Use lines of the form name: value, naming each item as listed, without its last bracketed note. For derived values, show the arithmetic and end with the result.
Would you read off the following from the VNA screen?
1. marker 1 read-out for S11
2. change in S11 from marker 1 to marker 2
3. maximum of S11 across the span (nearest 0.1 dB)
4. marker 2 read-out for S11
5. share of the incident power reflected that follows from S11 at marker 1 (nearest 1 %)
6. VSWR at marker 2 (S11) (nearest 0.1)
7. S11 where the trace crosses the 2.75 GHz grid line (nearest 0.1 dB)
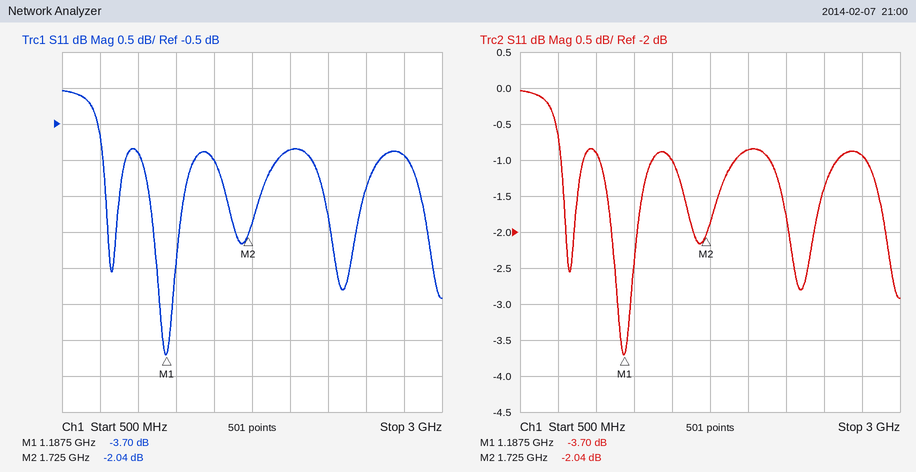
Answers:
marker 1 read-out for S11: -3.70 dB
change in S11 from marker 1 to marker 2: -2.04 − (-3.7) = 1.66 dB
maximum of S11 across the span: 0.0 dB
marker 2 read-out for S11: -2.04 dB
share of the incident power reflected that follows from S11 at marker 1: 10^(-3.7/10) ≈ 43 %
VSWR at marker 2 (S11): (1 + 0.7907)/(1 − 0.7907) ≈ 8.6
S11 where the trace crosses the 2.75 GHz grid line: -0.9 dB
